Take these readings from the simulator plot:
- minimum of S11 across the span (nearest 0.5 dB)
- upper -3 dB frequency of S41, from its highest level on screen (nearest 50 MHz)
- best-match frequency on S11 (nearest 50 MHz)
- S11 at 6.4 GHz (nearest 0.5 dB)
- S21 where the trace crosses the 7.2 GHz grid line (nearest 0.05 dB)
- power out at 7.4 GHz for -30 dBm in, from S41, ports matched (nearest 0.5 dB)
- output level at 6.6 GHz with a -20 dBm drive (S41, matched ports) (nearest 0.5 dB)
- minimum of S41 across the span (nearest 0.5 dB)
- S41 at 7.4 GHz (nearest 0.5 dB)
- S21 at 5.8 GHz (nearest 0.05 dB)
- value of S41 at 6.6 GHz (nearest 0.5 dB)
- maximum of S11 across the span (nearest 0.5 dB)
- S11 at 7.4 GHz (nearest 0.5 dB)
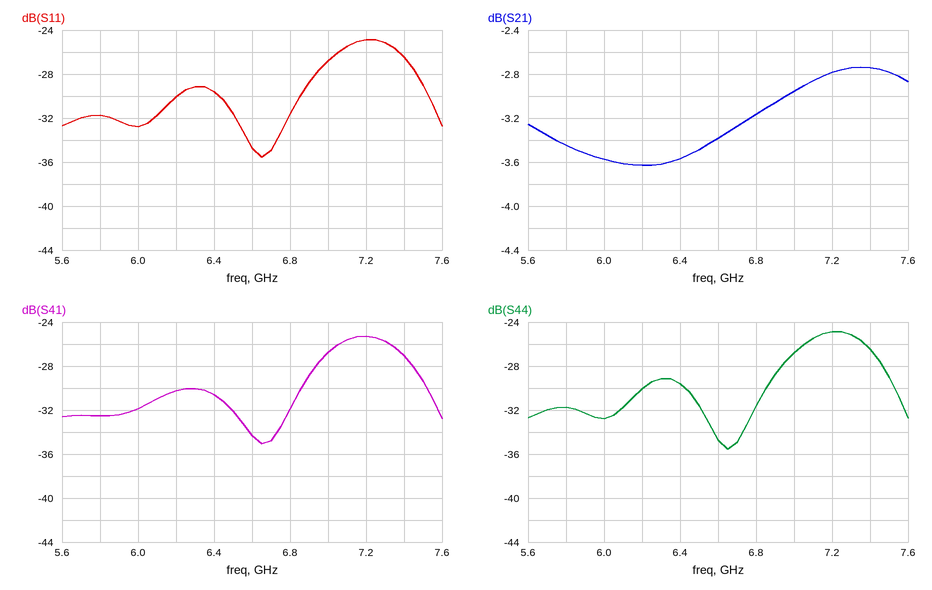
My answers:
-35.5 dB
7.45 GHz
6.65 GHz
-29.5 dB
-2.80 dB
-57.0 dBm
-54.5 dBm
-35.0 dB
-27.0 dB
-3.45 dB
-34.5 dB
-25.0 dB
-26.5 dB
